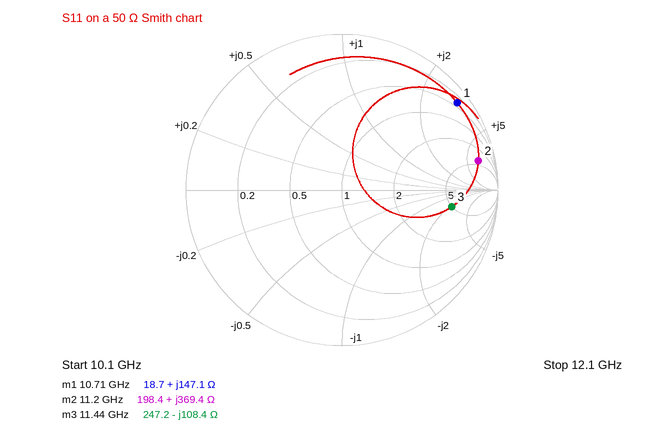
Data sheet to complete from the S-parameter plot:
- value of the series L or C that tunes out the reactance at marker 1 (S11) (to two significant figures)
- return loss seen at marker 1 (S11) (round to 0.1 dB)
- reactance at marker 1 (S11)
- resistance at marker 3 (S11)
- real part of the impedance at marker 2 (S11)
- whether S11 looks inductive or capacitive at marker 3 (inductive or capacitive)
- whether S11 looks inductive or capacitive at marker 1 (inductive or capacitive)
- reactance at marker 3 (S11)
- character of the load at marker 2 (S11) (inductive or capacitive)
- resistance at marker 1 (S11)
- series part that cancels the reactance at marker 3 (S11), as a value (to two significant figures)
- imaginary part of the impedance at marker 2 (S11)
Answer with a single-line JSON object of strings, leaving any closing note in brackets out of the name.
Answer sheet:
{"value of the series L or C that tunes out the reactance at marker 1 (S11)": "100 fF", "return loss seen at marker 1 (S11)": "0.7 dB", "reactance at marker 1": "+147.1 Ω", "resistance at marker 3": "247.2 Ω", "real part of the impedance at marker 2": "198.4 Ω", "whether S11 looks inductive or capacitive at marker 3": "capacitive", "whether S11 looks inductive or capacitive at marker 1": "inductive", "reactance at marker 3": "-108.4 Ω", "character of the load at marker 2 (S11)": "inductive", "resistance at marker 1": "18.7 Ω", "series part that cancels the reactance at marker 3 (S11), as a value": "1.5 nH", "imaginary part of the impedance at marker 2": "+369.4 Ω"}
